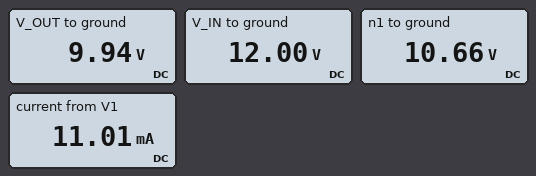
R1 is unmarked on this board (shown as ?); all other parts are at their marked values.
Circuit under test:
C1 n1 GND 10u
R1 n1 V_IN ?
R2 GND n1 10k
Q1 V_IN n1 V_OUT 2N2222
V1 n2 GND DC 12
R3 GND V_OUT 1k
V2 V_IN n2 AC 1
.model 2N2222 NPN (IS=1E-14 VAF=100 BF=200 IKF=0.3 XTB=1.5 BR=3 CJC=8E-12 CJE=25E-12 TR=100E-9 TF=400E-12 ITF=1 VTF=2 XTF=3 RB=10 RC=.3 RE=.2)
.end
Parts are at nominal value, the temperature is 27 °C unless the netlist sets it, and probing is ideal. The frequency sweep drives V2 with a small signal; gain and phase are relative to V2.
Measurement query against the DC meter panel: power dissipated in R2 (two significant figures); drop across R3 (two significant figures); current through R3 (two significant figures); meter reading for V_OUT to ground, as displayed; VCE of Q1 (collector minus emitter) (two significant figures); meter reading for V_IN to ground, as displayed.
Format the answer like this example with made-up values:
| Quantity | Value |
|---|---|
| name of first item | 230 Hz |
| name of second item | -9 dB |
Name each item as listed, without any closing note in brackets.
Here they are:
| Quantity | Value |
|---|---|
| power dissipated in R2 | 11 mW |
| drop across R3 | 9.9 V |
| current through R3 | 9.9 mA |
| meter reading for V_OUT to ground, as displayed | 9.94 V |
| VCE of Q1 (collector minus emitter) | 2.1 V |
| meter reading for V_IN to ground, as displayed | 12.00 V |
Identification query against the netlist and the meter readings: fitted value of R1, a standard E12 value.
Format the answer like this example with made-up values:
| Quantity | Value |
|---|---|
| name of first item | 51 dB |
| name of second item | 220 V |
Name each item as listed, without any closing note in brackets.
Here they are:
| Quantity | Value |
|---|---|
| fitted value of R1, a standard E12 value | 1.2 kΩ |
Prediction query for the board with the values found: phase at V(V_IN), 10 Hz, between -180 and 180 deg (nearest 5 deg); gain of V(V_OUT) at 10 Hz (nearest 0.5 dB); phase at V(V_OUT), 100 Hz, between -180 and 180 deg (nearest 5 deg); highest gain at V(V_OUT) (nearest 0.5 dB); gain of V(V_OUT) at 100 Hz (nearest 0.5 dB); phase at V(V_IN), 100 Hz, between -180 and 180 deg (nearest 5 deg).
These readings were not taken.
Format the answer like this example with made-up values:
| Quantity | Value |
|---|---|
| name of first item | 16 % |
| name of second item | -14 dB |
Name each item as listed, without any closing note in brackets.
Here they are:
| Quantity | Value |
|---|---|
| phase at V(V_IN), 10 Hz, between -180 and 180 deg | 0 deg |
| gain of V(V_OUT) at 10 Hz | -2.5 dB |
| phase at V(V_OUT), 100 Hz, between -180 and 180 deg | -80 deg |
| highest gain at V(V_OUT) | -1.0 dB |
| gain of V(V_OUT) at 100 Hz | -17.5 dB |
| phase at V(V_IN), 100 Hz, between -180 and 180 deg | 0 deg |
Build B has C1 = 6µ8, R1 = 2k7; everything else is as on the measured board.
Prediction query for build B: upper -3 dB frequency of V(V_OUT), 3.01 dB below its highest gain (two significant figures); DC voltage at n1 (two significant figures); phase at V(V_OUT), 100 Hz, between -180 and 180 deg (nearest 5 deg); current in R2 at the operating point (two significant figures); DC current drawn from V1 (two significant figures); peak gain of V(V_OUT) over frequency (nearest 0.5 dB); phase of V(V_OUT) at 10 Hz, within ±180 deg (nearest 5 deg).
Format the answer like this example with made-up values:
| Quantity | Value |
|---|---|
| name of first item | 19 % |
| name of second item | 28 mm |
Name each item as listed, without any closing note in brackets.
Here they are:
| Quantity | Value |
|---|---|
| upper -3 dB frequency of V(V_OUT), 3.01 dB below its highest gain | 11 Hz |
| DC voltage at n1 | 9.4 V |
| phase at V(V_OUT), 100 Hz, between -180 and 180 deg | -85 deg |
| current in R2 at the operating point | 940 µA |
| DC current drawn from V1 | 9.6 mA |
| peak gain of V(V_OUT) over frequency | -2.0 dB |
| phase of V(V_OUT) at 10 Hz, within ±180 deg | -40 deg |
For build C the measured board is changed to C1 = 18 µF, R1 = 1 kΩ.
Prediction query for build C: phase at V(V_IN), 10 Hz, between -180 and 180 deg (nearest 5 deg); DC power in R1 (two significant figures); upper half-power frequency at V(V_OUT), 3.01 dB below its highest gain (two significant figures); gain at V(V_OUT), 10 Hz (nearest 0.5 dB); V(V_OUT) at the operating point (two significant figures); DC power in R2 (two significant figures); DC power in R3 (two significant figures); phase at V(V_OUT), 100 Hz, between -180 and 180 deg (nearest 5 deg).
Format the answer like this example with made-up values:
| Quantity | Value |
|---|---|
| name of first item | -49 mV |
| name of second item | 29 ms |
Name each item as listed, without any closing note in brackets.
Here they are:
| Quantity | Value |
|---|---|
| phase at V(V_IN), 10 Hz, between -180 and 180 deg | 0 deg |
| DC power in R1 | 1.3 mW |
| upper half-power frequency at V(V_OUT), 3.01 dB below its highest gain | 9.8 Hz |
| gain at V(V_OUT), 10 Hz | -4.0 dB |
| V(V_OUT) at the operating point | 10 V |
| DC power in R2 | 12 mW |
| DC power in R3 | 100 mW |
| phase at V(V_OUT), 100 Hz, between -180 and 180 deg | -85 deg |
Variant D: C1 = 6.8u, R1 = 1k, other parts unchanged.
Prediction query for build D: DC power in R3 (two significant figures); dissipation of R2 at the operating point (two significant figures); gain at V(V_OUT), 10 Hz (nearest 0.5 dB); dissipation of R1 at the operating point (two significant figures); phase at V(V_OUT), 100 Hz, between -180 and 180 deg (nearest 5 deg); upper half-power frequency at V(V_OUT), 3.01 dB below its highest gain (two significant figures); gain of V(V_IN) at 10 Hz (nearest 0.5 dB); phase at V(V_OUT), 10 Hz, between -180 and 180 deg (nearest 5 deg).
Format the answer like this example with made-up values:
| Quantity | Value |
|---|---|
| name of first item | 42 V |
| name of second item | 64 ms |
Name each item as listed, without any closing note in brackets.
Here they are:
| Quantity | Value |
|---|---|
| DC power in R3 | 100 mW |
| dissipation of R2 at the operating point | 12 mW |
| gain at V(V_OUT), 10 Hz | -1.5 dB |
| dissipation of R1 at the operating point | 1.3 mW |
| phase at V(V_OUT), 100 Hz, between -180 and 180 deg | -75 deg |
| upper half-power frequency at V(V_OUT), 3.01 dB below its highest gain | 26 Hz |
| gain of V(V_IN) at 10 Hz | 0 dB |
| phase at V(V_OUT), 10 Hz, between -180 and 180 deg | -20 deg |
